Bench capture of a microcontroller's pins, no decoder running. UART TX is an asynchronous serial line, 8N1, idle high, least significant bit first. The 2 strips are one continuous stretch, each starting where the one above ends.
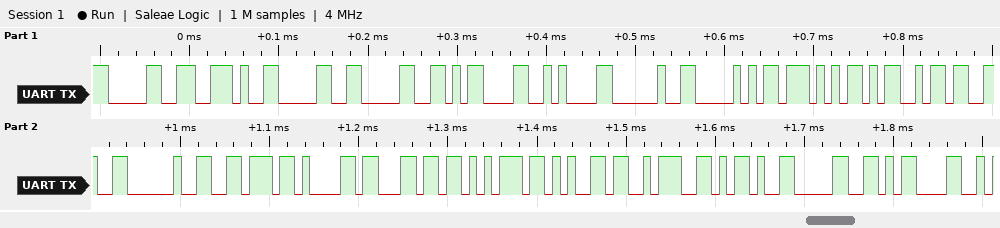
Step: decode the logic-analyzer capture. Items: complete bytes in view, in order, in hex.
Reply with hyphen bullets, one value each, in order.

- 30 2E 30 30 0D 0A 20 50 57 4D 33 20 76 61 6C 75 65 3A 2D 30 0D
